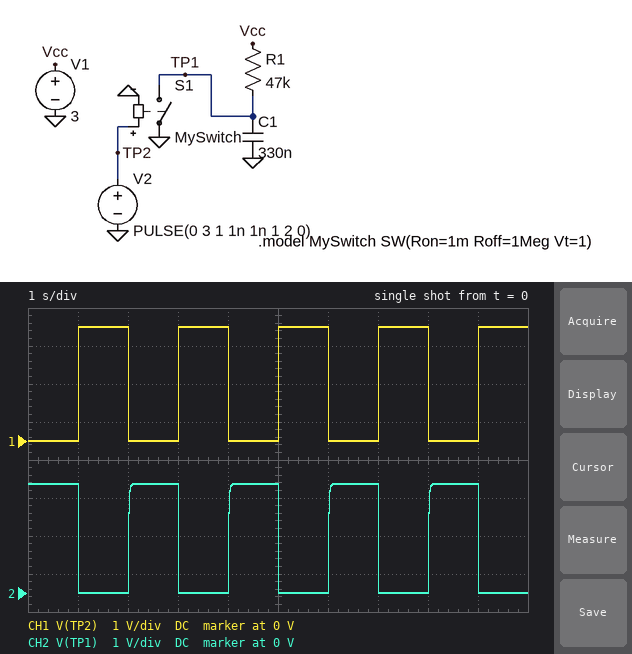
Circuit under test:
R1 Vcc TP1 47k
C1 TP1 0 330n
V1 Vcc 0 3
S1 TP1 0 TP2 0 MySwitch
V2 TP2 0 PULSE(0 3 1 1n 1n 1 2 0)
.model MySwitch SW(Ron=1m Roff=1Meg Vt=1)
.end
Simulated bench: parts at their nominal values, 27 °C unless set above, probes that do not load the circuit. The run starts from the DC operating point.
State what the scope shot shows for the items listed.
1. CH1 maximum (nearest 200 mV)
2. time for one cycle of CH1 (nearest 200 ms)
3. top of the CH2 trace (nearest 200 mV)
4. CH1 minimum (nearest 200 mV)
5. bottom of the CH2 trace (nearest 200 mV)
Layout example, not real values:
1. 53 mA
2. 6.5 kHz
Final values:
1. 3.0 V
2. 2.0 s
3. 2.8 V
4. 0 V
5. 0 V
